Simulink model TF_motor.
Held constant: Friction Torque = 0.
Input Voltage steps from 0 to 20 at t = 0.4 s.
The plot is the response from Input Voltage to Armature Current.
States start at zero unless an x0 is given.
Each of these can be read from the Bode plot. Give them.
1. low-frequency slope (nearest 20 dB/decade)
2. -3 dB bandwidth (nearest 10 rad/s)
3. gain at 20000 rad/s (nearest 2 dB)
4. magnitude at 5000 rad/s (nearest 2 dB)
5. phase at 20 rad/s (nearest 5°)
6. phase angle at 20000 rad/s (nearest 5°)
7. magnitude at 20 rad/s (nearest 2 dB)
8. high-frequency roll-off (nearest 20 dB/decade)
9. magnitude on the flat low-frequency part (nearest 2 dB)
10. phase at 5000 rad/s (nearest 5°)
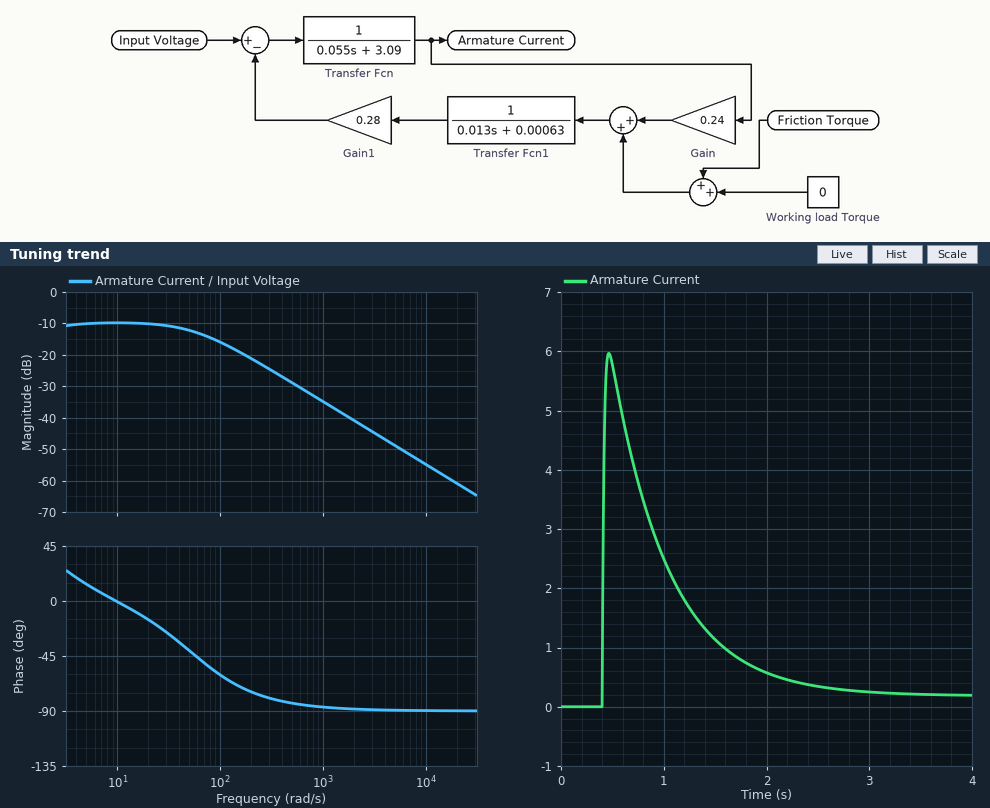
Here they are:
0 dB/decade
60 rad/s
-60 dB
-48 dB
-15°
-90°
-10 dB
-20 dB/decade
-10 dB
-90°
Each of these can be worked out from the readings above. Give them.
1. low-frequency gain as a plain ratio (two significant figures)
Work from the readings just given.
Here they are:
0.32
